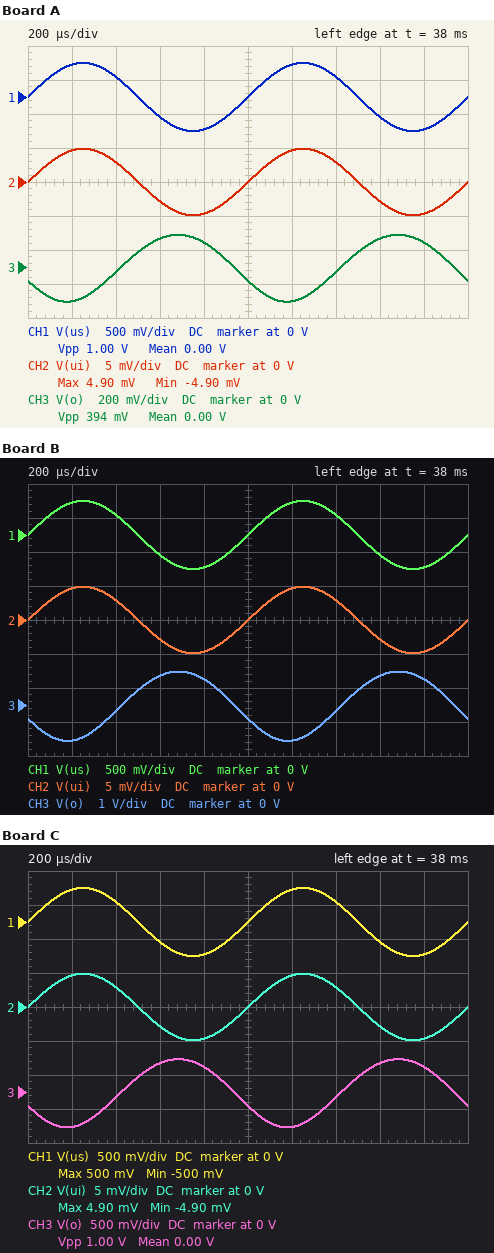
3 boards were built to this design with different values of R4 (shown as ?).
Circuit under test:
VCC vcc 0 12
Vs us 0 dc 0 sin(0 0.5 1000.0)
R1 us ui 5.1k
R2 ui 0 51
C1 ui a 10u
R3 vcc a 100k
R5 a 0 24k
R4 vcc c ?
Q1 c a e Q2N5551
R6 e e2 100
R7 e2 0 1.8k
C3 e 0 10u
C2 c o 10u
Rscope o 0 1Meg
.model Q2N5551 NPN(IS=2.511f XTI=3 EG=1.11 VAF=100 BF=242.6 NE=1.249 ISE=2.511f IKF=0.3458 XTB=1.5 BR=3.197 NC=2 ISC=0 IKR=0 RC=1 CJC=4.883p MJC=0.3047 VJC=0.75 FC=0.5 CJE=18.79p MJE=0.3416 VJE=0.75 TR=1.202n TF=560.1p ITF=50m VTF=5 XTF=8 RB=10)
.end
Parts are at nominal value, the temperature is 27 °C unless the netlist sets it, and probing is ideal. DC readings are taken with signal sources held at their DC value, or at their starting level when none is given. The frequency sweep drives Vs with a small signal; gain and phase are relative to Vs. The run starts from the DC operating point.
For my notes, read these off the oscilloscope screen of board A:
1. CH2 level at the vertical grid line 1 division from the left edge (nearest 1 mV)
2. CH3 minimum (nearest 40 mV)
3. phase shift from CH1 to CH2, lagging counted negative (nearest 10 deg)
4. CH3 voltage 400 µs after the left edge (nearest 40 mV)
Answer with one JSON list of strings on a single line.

["5 mV", "-200 mV", "0 deg", "-40 mV"]
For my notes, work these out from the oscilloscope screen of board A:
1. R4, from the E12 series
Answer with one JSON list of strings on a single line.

["1.5 kΩ"]
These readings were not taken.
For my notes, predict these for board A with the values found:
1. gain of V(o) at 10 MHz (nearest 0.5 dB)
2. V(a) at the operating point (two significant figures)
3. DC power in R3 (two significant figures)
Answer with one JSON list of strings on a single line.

["-9.0 dB", "2.2 V", "960 µW"]
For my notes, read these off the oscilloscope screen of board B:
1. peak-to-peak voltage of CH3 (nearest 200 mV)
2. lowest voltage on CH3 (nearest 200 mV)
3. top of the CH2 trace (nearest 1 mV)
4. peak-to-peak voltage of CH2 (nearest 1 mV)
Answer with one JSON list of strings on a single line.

["2.0 V", "-1.0 V", "5 mV", "10 mV"]
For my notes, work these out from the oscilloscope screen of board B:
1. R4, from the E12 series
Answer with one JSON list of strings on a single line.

["8.2 kΩ"]
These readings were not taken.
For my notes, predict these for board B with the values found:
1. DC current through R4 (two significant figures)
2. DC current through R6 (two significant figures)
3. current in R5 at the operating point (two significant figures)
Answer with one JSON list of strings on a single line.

["780 µA", "790 µA", "91 µA"]
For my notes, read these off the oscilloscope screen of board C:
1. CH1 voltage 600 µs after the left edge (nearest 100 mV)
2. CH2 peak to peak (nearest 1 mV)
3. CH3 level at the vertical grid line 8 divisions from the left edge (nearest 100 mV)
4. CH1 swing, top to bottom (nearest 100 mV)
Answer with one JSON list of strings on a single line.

["-300 mV", "10 mV", "400 mV", "1.0 V"]
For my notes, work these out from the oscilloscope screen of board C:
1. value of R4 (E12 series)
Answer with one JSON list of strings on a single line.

["3.9 kΩ"]
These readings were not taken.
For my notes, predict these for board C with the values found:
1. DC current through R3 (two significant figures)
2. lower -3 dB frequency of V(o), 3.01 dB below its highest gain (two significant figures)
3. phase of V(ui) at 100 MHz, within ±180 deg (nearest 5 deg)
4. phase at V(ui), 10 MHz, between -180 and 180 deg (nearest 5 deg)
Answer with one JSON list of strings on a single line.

["98 µA", "480 Hz", "-20 deg", "-25 deg"]
